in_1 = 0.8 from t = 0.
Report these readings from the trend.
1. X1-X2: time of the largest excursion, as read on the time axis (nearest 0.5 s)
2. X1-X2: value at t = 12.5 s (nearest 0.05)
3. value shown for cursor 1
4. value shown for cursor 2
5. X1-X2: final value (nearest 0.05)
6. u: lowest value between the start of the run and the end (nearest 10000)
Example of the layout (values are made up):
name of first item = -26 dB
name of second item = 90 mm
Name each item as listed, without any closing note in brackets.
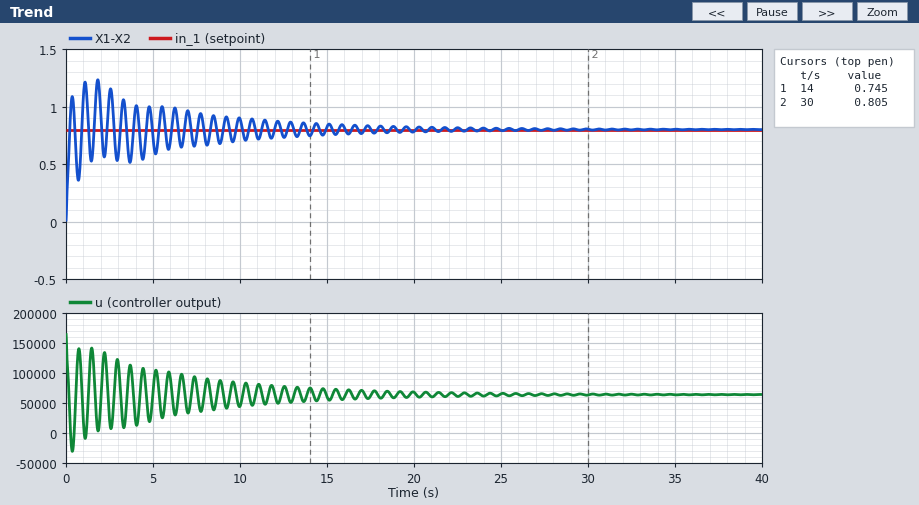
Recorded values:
X1-X2: time of the largest excursion, as read on the time axis = 2.0 s
X1-X2: value at t = 12.5 s = 0.75
value shown for cursor 1 = 0.745
value shown for cursor 2 = 0.805
X1-X2: final value = 0.80
u: lowest value between the start of the run and the end = -30000
